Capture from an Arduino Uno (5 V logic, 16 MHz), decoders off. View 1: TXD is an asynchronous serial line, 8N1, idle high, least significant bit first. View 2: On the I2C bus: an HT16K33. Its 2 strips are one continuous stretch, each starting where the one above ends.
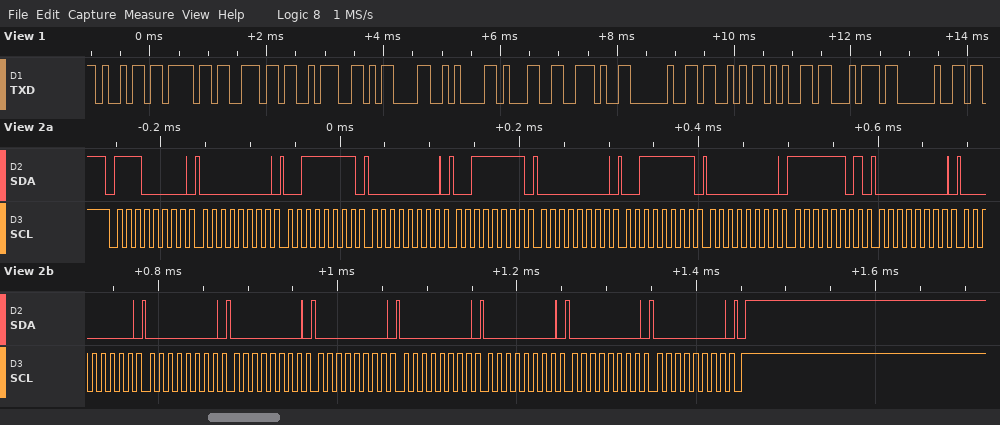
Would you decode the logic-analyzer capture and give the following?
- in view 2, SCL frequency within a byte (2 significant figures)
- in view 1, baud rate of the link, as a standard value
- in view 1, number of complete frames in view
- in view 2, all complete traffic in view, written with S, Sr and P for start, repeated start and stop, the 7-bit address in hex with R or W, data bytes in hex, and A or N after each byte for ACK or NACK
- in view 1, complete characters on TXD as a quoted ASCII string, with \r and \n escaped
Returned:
100 kHz
9600 baud
13
S 70W A 00 A 3F A 00 A 3F A 00 A 3F A 00 A FD A 00 A 00 A 00 A 00 A 00 A 00 A 00 A 00 A 00 A P
"ion:\r\n1. Set "
